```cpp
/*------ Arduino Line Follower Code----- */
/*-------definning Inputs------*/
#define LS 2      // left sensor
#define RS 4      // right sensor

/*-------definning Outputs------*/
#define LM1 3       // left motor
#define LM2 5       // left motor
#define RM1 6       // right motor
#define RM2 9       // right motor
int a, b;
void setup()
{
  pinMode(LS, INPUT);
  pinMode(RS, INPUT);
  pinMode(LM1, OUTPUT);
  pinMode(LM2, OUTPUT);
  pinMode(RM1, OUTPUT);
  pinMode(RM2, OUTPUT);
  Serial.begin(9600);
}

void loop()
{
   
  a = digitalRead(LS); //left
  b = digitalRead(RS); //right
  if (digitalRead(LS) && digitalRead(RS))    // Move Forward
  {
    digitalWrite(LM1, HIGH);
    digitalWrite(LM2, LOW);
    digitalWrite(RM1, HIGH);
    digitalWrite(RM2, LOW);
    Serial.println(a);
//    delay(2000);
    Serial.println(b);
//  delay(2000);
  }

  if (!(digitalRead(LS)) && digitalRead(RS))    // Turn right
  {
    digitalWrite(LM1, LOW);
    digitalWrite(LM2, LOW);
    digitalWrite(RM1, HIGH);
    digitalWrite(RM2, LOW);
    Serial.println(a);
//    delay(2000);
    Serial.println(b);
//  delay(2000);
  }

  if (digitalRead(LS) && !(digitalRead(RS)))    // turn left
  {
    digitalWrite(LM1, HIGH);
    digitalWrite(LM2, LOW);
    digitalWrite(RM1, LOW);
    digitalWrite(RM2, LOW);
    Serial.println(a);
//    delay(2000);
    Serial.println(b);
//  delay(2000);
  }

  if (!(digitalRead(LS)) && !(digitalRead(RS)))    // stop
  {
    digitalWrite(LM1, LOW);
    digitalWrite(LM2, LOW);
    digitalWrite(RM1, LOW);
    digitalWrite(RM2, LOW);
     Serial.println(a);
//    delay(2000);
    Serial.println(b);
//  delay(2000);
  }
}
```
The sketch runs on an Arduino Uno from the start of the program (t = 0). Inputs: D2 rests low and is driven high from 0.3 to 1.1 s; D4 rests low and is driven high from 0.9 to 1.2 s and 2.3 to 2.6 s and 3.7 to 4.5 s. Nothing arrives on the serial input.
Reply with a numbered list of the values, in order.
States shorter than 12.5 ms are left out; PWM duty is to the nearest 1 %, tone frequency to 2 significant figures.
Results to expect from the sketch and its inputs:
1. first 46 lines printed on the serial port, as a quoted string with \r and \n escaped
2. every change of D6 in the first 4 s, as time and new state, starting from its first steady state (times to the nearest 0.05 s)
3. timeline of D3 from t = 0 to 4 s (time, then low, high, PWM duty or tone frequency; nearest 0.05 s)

1. "0\r\n0\r\n0\r\n0\r\n0\r\n0\r\n0\r\n0\r\n0\r\n0\r\n0\r\n0\r\n0\r\n0\r\n0\r\n0\r\n0\r\n0\r\n0\r\n0\r\n0\r\n0\r\n0\r\n0\r\n0\r\n0\r\n0\r\n0\r\n0\r\n0\r\n0\r\n0\r\n0\r\n0\r\n0\r\n0\r\n0\r\n0\r\n0\r\n0\r\n0\r\n0\r\n0\r\n0\r\n0\r\n0\r\n"
2. 0 s low; 0.9 s high; 1.2 s low; 2.3 s high; 2.6 s low; 3.7 s high
3. 0 s low; 0.3 s high; 1.1 s low
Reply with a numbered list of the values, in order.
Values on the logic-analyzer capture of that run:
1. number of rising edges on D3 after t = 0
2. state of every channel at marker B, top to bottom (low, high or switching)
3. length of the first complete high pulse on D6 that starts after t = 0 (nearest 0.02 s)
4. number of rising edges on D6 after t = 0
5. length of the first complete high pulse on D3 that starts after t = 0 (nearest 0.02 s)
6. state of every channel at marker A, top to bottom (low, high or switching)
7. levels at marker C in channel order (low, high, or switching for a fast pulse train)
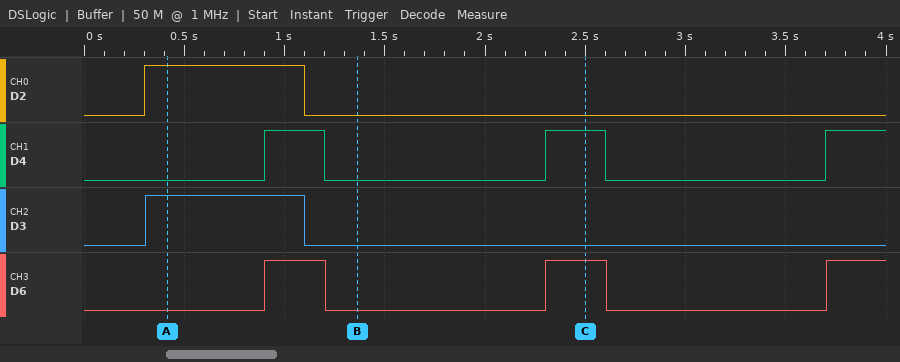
1. 1
2. D2 low, D4 low, D3 low, D6 low
3. 0.30 s
4. 3
5. 0.80 s
6. D2 high, D4 low, D3 high, D6 low
7. D2 low, D4 high, D3 low, D6 high
